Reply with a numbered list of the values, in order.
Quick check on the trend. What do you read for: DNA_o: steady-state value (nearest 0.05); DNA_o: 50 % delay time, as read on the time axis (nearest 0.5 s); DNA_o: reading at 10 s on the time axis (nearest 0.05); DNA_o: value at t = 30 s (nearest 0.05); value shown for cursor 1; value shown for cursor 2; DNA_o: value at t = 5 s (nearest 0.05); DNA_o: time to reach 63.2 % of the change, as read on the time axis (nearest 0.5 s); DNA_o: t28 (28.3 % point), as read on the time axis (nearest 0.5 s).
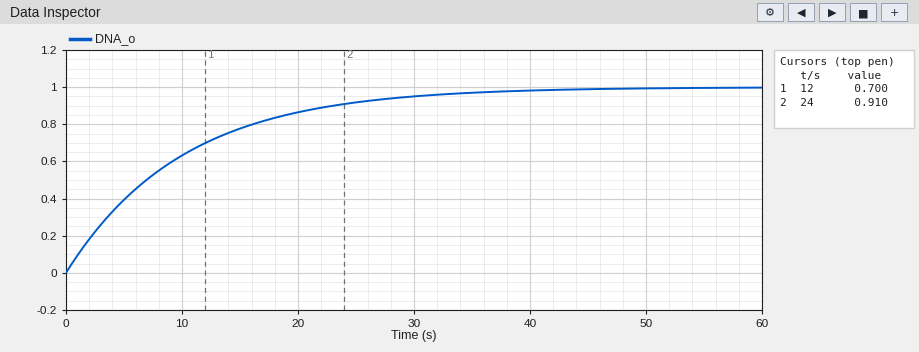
1. 1.00
2. 7.0 s
3. 0.65
4. 0.95
5. 0.700
6. 0.910
7. 0.40
8. 10.0 s
9. 3.5 s
